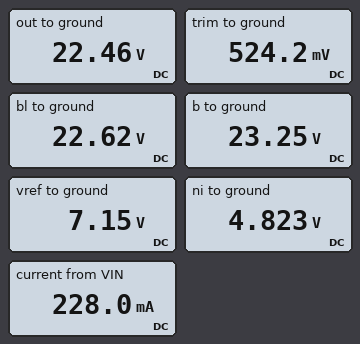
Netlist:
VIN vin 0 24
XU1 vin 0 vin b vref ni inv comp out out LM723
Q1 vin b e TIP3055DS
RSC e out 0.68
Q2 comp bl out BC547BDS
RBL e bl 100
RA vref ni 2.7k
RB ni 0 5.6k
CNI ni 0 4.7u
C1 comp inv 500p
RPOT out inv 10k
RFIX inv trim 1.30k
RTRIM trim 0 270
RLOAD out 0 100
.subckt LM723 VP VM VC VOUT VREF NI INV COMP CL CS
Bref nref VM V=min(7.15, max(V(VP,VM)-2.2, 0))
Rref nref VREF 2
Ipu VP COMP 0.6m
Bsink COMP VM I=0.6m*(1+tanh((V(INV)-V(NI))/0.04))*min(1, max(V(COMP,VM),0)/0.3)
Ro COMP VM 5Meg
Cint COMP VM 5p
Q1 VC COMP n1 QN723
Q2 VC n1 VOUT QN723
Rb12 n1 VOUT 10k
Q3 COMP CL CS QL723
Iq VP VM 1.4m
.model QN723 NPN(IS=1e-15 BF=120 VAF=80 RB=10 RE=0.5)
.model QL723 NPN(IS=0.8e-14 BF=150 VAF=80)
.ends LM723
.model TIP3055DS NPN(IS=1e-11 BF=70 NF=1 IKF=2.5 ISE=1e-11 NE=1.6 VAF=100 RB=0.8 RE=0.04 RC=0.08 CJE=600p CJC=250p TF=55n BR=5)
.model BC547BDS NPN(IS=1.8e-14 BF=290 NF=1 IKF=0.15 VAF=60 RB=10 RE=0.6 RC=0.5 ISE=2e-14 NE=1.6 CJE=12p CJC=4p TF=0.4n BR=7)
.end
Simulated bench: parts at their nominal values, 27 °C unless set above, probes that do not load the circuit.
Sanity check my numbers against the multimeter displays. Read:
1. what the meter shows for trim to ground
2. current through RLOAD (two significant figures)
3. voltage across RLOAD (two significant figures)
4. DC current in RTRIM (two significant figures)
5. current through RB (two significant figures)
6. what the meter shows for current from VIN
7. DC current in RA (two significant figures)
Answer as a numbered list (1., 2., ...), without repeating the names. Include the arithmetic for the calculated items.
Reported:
1. 524.2 mV
2. (22.46 V) / 100 Ω = 220 mA
3. 22.46 V = 22 V
4. (524.2 mV) / 270 Ω = 1.9 mA
5. (4.823 V) / 5.6 kΩ = 860 µA
6. 228.0 mA
7. (7.15 V - 4.823 V) / 2.7 kΩ = 860 µA
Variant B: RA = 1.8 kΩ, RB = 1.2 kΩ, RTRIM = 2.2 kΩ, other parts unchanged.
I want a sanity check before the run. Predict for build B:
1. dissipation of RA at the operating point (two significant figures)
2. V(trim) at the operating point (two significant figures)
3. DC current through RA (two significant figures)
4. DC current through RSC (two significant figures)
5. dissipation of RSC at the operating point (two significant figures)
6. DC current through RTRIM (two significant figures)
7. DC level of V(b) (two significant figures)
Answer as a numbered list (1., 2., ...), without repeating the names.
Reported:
1. 10 mW
2. 1.8 V
3. 2.4 mA
4. 110 mA
5. 8.4 mW
6. 820 µA
7. 12 V
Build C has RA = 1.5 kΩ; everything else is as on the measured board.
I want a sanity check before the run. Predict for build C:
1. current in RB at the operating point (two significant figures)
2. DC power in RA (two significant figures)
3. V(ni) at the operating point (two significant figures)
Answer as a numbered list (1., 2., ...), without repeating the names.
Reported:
1. 1.0 mA
2. 1.5 mW
3. 5.6 V
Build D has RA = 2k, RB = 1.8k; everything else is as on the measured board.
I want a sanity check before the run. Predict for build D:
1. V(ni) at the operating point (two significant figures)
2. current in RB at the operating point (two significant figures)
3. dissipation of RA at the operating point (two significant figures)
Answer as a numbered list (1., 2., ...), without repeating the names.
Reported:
1. 3.4 V
2. 1.9 mA
3. 7.1 mW
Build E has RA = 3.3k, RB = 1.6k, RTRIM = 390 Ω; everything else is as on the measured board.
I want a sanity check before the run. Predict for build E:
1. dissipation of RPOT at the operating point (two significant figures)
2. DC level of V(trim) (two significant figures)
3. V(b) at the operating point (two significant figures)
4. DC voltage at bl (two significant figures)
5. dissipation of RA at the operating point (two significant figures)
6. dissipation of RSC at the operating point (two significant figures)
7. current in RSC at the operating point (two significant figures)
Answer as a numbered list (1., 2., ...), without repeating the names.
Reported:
1. 19 mW
2. 540 mV
3. 17 V
4. 16 V
5. 7.0 mW
6. 18 mW
7. 160 mA
